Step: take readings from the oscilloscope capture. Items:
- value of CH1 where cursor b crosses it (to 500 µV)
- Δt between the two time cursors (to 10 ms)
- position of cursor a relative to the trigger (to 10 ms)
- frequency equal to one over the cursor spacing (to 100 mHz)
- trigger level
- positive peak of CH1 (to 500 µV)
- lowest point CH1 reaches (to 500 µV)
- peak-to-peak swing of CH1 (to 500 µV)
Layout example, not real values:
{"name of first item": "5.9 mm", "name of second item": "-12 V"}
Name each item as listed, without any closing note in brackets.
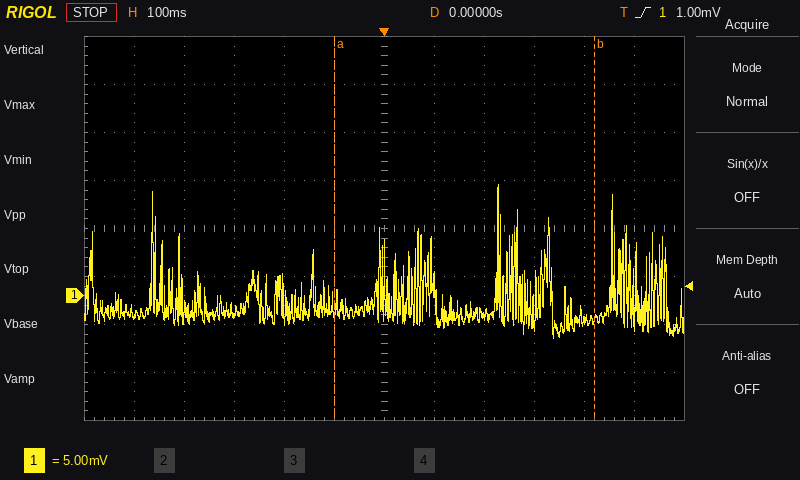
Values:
{"value of CH1 where cursor b crosses it": "-2.5 mV", "Δt between the two time cursors": "520 ms", "position of cursor a relative to the trigger": "-100 ms", "frequency equal to one over the cursor spacing": "1.9 Hz", "trigger level": "1.00 mV", "positive peak of CH1": "11.5 mV", "lowest point CH1 reaches": "-4.5 mV", "peak-to-peak swing of CH1": "16.0 mV"}
